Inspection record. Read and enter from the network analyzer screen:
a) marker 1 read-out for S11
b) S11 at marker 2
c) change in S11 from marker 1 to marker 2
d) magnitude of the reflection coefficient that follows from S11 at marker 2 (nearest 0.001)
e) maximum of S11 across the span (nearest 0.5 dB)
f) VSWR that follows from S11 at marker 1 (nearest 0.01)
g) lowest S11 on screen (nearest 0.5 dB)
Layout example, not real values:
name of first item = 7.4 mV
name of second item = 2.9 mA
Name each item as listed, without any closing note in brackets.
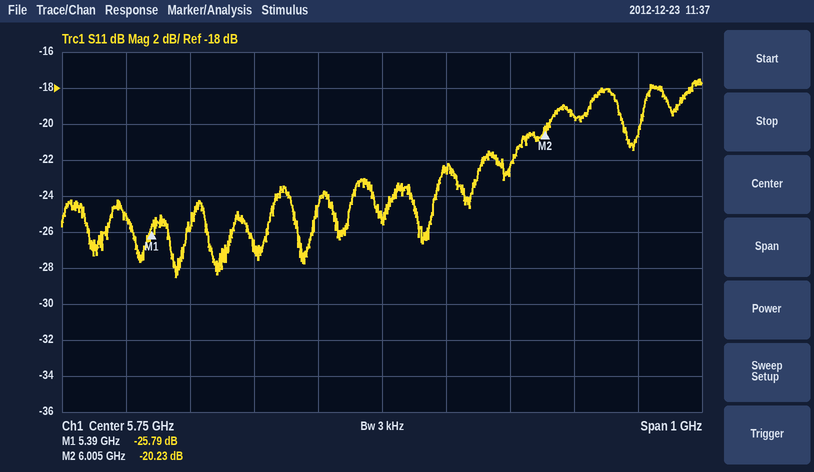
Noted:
marker 1 read-out for S11 = -25.79 dB
S11 at marker 2 = -20.23 dB
change in S11 from marker 1 to marker 2 = 5.56 dB
magnitude of the reflection coefficient that follows from S11 at marker 2 = 0.097
maximum of S11 across the span = -17.5 dB
VSWR that follows from S11 at marker 1 = 1.11
lowest S11 on screen = -28.5 dB
